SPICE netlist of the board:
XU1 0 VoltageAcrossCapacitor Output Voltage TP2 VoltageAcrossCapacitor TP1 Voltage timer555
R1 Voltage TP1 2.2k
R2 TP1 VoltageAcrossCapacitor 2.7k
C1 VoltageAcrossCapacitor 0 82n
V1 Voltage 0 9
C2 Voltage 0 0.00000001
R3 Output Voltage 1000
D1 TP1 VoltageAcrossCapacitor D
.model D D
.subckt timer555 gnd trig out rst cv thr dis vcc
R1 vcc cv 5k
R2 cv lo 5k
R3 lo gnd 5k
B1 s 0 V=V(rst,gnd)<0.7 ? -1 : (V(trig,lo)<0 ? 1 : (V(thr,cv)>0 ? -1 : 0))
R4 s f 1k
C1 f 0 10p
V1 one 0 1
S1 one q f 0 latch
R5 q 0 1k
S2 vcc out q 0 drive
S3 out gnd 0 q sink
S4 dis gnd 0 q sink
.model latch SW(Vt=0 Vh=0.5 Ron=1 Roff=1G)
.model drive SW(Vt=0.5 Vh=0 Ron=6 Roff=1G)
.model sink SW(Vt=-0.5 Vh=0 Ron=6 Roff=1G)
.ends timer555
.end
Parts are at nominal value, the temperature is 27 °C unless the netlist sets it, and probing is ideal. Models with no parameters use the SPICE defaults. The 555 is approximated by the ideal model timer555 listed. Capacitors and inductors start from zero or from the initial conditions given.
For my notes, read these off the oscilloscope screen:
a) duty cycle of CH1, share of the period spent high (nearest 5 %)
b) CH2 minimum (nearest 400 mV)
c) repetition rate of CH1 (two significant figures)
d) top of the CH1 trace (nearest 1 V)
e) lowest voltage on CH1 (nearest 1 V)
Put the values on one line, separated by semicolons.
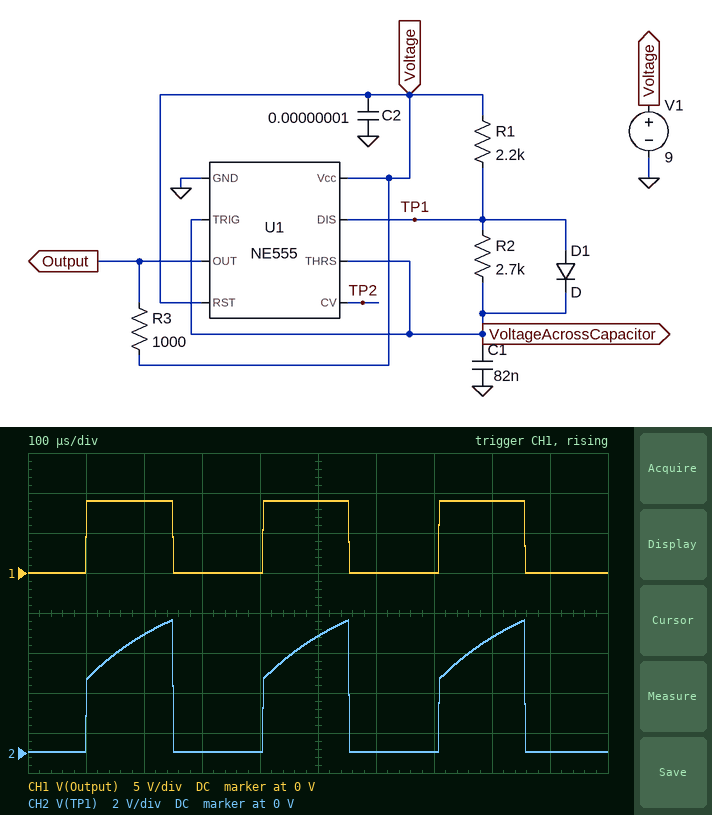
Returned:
50 %; 0 V; 3.3 kHz; 9 V; 0 V
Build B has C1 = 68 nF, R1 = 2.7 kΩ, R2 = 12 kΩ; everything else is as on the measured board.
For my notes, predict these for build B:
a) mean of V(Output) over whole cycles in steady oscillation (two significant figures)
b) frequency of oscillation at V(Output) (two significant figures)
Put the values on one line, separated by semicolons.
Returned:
1.9 V; 1.4 kHz
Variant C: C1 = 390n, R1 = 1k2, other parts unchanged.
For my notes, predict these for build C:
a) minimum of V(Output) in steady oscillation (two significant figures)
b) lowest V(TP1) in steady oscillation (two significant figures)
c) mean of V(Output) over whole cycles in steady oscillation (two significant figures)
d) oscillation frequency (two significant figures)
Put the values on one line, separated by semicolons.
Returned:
54 mV; 51 mV; 3.1 V; 890 Hz
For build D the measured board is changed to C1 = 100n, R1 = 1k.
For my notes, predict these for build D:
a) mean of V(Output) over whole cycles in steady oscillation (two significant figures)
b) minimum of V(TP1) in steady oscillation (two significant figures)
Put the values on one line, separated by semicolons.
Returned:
2.8 V; 60 mV
